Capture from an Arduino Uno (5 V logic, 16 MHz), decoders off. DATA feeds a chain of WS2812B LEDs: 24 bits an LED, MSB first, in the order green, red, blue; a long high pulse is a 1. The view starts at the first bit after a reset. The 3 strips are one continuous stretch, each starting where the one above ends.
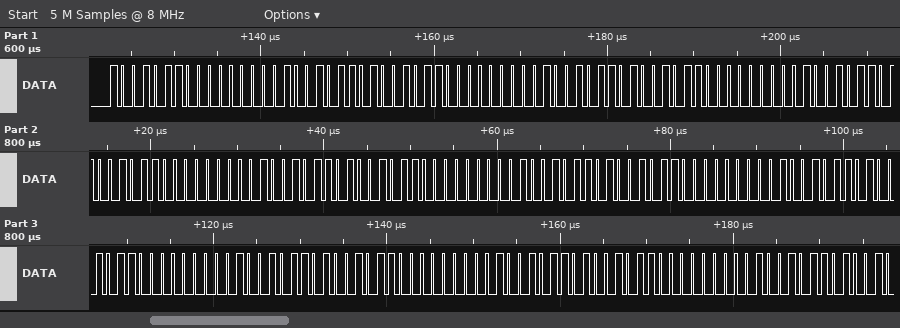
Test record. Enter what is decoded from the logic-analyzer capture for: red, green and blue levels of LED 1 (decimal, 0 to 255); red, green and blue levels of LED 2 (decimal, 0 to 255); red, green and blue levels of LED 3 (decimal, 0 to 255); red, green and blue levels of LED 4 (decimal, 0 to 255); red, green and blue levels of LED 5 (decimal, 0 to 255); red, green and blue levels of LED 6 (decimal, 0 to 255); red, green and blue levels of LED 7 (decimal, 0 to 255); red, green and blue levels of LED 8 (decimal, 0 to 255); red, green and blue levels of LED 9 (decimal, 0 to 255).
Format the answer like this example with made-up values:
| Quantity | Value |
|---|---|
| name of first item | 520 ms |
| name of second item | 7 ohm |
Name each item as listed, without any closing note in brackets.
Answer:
| Quantity | Value |
|---|---|
| red, green and blue levels of LED 1 | 0, 150, 150 |
| red, green and blue levels of LED 2 | 0, 150, 150 |
| red, green and blue levels of LED 3 | 0, 150, 150 |
| red, green and blue levels of LED 4 | 0, 150, 150 |
| red, green and blue levels of LED 5 | 0, 150, 150 |
| red, green and blue levels of LED 6 | 0, 150, 150 |
| red, green and blue levels of LED 7 | 0, 150, 150 |
| red, green and blue levels of LED 8 | 0, 150, 150 |
| red, green and blue levels of LED 9 | 0, 150, 150 |
